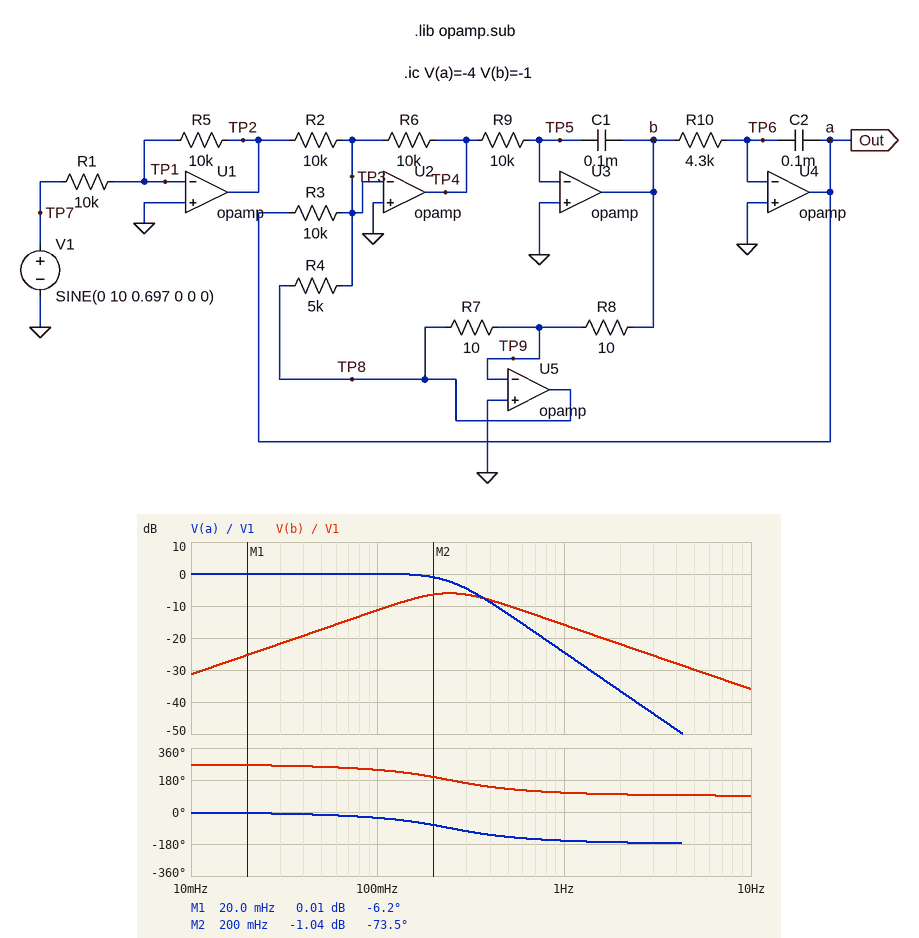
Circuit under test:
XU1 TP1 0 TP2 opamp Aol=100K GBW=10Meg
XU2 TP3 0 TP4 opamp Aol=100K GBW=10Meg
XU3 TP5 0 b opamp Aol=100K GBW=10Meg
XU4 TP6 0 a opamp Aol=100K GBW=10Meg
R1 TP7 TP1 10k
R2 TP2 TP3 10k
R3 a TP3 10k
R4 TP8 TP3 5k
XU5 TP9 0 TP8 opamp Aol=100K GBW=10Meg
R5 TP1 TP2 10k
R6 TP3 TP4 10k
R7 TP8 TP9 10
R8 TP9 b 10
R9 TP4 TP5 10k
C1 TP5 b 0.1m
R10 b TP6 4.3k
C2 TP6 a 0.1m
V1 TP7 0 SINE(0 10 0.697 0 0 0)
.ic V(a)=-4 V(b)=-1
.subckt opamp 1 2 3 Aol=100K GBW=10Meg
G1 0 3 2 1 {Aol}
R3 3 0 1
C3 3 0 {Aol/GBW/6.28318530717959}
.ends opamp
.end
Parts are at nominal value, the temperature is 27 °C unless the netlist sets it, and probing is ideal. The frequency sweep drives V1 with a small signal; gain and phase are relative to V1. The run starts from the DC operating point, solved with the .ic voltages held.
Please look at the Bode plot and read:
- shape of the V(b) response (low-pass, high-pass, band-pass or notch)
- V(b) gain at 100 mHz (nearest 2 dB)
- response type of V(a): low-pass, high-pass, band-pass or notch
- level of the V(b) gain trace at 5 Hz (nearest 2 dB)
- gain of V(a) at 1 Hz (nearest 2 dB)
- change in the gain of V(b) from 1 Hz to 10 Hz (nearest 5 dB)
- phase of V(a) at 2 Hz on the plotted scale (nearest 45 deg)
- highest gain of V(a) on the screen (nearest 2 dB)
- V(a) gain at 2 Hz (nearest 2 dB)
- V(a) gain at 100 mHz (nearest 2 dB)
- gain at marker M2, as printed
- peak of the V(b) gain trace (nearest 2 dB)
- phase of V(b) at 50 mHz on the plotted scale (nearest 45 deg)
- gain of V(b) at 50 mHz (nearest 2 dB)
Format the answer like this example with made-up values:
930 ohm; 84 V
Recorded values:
band-pass; -12 dB; low-pass; -30 dB; -24 dB; -20 dB; -180 deg; 0 dB; -36 dB; 0 dB; -1.04 dB; -6 dB; 270 deg; -18 dB
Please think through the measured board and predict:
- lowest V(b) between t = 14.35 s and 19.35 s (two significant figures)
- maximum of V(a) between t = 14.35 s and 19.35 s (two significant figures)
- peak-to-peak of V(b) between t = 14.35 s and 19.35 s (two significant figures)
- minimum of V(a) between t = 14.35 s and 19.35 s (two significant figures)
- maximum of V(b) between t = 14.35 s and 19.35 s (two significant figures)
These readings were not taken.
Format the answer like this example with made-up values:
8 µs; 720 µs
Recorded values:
-2.3 V; 1.2 V; 4.6 V; -1.2 V; 2.3 V
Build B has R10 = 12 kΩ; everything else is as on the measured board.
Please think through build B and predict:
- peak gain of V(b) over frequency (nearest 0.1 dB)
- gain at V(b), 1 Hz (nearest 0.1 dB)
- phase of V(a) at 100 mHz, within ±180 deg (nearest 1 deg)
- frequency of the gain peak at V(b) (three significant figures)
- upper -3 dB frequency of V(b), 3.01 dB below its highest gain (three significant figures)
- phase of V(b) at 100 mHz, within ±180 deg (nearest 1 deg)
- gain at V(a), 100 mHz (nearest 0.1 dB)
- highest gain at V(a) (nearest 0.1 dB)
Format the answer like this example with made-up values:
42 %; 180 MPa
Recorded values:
-6.0 dB; -16.2 dB; -71 deg; 145 mHz; 375 mHz; -161 deg; -4.1 dB; 0 dB
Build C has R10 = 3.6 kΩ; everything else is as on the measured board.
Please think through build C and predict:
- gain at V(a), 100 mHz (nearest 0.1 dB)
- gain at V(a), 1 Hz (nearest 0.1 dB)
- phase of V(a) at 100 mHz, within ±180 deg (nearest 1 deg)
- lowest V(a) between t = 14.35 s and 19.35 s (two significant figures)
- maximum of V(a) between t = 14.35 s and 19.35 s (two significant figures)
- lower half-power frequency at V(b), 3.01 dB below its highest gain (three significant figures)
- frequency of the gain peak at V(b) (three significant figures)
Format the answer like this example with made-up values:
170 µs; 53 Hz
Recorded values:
0.3 dB; -22.9 dB; -28 deg; -1.5 V; 1.5 V; 150 mHz; 265 mHz
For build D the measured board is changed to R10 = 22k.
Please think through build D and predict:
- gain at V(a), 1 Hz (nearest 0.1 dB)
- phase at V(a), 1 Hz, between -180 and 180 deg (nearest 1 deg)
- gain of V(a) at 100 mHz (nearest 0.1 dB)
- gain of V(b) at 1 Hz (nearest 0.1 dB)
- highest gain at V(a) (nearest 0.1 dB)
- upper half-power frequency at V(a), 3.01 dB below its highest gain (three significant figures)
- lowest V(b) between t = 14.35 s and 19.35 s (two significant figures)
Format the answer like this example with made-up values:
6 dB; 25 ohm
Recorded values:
-39.1 dB; -162 deg; -8.8 dB; -16.3 dB; 0 dB; 40.7 mHz; -2.1 V
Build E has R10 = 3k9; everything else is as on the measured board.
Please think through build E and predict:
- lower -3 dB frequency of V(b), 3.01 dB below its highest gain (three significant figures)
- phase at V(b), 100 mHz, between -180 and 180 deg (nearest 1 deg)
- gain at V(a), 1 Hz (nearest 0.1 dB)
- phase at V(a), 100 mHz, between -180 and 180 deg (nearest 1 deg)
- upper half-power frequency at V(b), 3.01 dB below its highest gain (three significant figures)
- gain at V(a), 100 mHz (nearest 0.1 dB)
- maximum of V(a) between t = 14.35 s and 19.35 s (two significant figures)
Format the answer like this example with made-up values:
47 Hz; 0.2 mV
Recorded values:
141 mHz; -120 deg; -23.6 dB; -30 deg; 460 mHz; 0.2 dB; 1.4 V
